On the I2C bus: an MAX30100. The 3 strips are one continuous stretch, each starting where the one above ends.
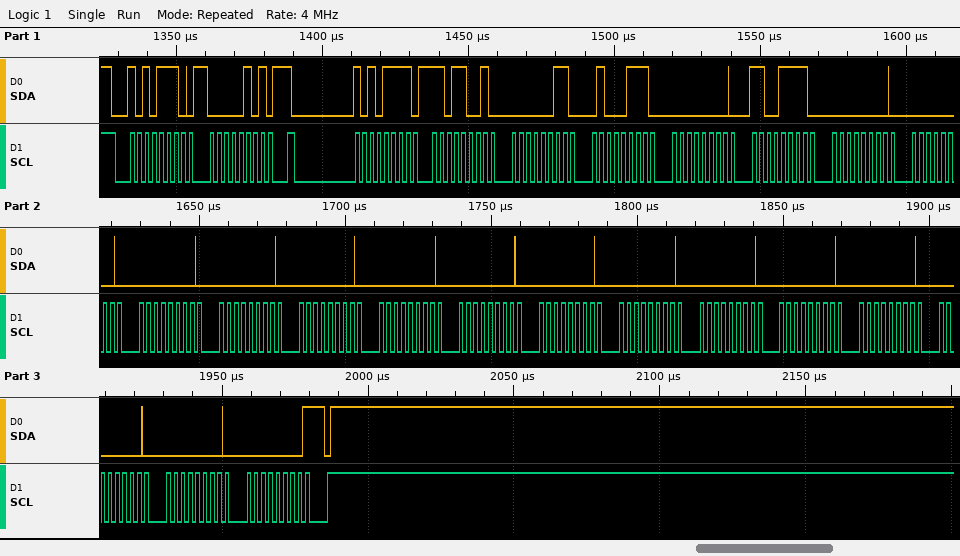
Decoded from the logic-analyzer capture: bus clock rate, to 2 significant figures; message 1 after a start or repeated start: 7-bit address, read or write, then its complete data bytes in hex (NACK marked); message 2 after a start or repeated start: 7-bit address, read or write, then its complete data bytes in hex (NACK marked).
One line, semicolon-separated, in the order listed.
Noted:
400 kHz; 0x57 write: 05; 0x57 read: D9 03 47 00 CF 00 00 00 00 00 00 00 00 00 00 00 00 00 00 00 NACK
